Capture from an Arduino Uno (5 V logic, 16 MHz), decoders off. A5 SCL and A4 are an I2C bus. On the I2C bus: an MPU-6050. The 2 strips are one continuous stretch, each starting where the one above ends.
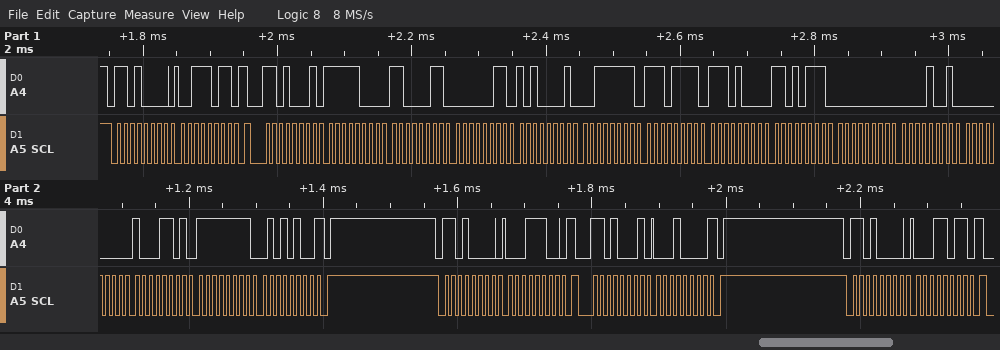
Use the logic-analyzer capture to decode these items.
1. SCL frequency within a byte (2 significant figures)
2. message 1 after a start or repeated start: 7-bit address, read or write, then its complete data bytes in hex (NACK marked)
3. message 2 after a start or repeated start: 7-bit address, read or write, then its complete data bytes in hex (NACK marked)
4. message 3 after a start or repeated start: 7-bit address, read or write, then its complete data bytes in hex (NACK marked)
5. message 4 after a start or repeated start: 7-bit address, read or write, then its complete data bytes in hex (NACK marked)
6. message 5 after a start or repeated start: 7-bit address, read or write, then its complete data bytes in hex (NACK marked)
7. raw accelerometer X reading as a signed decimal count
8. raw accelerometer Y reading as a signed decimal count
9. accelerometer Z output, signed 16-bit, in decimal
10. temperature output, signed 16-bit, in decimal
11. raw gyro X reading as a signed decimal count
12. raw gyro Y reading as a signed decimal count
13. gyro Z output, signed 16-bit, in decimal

100 kHz
0x68 write: 3B
0x68 read: F8 C3 03 A1 3F EF E8 D7 00 09 00 8D FF 54 NACK
0x68 write: 1C
0x68 read: 10 NACK
0x68 write: 1B
-1853
929
16367
-5929
9
141
-172
